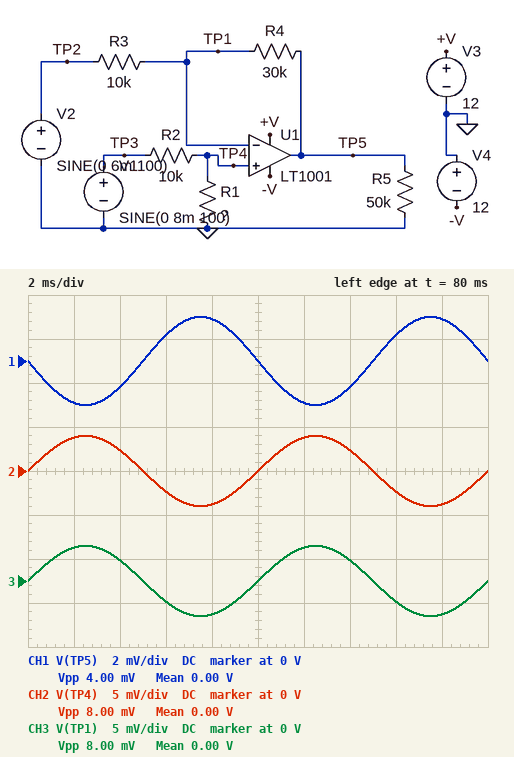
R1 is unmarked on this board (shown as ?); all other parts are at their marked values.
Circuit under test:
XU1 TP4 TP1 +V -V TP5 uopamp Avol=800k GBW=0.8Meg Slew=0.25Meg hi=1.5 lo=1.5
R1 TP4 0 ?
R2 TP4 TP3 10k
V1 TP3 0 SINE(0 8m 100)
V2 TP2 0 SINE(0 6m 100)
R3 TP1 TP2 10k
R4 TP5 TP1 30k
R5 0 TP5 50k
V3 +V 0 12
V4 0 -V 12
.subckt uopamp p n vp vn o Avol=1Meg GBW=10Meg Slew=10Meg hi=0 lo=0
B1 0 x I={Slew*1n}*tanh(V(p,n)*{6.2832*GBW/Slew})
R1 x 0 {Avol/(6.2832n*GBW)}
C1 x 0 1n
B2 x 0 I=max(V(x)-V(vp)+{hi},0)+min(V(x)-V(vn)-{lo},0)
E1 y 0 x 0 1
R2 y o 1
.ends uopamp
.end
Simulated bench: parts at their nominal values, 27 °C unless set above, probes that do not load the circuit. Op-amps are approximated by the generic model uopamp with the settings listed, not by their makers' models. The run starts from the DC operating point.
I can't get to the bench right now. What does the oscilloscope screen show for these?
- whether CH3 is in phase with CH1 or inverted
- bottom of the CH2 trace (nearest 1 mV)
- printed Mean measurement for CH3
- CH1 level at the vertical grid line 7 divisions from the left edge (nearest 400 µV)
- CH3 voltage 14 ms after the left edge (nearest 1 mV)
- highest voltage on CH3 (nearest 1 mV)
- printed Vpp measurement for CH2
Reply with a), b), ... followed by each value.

a) inverted
b) -4 mV
c) 0.00 V
d) -1.2 mV
e) 2 mV
f) 4 mV
g) 8.00 mV
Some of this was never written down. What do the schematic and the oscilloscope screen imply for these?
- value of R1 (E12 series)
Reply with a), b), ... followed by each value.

a) 10 kΩ
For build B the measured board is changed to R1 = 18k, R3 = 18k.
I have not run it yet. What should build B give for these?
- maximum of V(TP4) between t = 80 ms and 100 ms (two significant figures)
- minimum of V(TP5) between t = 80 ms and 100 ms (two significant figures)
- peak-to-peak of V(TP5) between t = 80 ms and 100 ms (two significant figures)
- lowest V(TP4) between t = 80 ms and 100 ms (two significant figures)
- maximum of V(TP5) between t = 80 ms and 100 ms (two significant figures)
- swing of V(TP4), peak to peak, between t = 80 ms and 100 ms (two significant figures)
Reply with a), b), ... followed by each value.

a) 5.1 mV
b) -3.7 mV
c) 7.4 mV
d) -5.1 mV
e) 3.7 mV
f) 10 mV
